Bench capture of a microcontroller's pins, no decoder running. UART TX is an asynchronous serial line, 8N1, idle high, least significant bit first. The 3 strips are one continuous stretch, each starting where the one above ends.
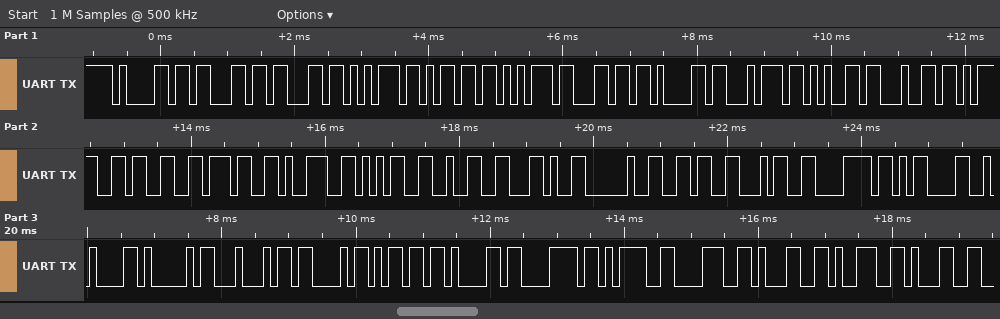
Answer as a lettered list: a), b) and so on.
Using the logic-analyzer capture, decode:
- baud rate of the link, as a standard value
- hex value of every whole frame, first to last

a) 9600 baud
b) 61 63 63 75 6D 75 6C 61 74 65 64 3D 33 37 39 35 32 2C 20 36 34 78 0D 0A 41 44 43 6D 61 78 3D 38 31 39 31
